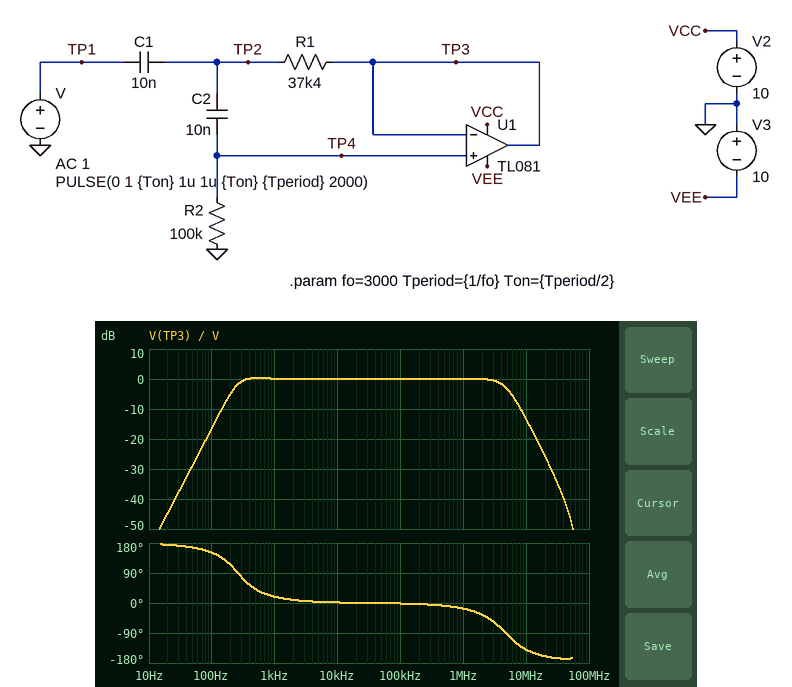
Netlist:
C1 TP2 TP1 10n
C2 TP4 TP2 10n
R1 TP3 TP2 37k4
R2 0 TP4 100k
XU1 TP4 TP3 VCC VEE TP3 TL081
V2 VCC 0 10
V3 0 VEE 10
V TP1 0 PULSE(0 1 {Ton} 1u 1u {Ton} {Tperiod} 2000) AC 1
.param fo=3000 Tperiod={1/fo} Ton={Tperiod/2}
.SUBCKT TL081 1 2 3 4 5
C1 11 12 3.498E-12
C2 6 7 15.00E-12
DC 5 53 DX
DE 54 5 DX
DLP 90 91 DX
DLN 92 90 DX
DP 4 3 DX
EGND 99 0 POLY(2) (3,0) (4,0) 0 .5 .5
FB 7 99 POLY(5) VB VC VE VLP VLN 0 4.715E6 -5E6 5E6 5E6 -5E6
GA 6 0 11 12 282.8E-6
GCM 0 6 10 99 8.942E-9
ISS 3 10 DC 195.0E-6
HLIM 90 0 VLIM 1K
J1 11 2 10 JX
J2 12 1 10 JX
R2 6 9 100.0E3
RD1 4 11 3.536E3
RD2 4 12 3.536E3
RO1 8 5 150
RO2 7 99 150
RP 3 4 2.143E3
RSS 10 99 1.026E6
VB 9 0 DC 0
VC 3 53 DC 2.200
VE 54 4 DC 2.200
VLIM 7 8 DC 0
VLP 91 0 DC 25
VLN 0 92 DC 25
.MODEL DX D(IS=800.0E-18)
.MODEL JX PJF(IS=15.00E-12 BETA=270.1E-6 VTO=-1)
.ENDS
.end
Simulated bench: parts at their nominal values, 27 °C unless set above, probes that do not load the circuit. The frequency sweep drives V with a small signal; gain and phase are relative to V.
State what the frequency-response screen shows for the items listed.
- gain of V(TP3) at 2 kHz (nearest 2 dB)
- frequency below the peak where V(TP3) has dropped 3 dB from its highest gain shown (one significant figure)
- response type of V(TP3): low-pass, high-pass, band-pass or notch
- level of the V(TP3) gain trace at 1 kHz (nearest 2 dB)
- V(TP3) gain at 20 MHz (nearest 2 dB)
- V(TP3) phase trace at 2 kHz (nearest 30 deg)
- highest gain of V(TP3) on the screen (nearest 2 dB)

0 dB
200 Hz
band-pass
0 dB
-26 dB
0 deg
0 dB
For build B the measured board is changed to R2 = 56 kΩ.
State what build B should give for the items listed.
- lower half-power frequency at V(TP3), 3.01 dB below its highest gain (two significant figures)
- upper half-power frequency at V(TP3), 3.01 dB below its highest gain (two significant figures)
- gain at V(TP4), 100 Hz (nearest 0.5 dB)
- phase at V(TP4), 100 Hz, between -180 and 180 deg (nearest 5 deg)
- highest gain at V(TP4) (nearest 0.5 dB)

410 Hz
4.8 MHz
-22.0 dB
155 deg
0 dB
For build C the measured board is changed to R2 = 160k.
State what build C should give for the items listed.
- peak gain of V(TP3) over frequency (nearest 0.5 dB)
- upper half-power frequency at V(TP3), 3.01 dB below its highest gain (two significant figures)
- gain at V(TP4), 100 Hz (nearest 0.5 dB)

1.5 dB
4.0 MHz
-11.5 dB
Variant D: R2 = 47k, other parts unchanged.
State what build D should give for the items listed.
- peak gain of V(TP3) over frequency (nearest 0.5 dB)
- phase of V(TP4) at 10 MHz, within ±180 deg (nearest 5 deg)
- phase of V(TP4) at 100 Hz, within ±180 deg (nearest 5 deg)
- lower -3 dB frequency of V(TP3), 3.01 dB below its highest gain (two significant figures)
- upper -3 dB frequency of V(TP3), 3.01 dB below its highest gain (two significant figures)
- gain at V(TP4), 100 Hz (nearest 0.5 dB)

0 dB
0 deg
155 deg
500 Hz
4.8 MHz
-23.5 dB
